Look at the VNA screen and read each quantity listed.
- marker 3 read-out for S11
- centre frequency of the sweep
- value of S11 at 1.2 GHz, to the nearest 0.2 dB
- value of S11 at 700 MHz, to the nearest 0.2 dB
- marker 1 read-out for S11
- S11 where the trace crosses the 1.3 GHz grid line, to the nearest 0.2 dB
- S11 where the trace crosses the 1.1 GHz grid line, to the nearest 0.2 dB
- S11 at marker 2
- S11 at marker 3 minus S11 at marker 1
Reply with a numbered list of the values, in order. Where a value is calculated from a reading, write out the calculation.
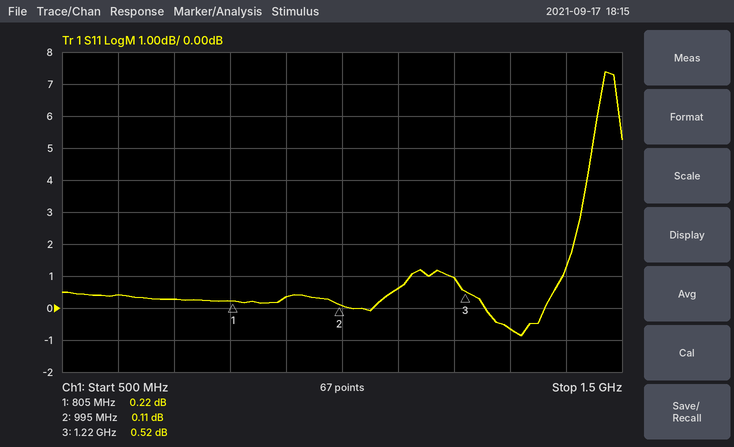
1. 0.52 dB
2. 1 GHz
3. 1.0 dB
4. 0.2 dB
5. 0.22 dB
6. -0.6 dB
7. 0.6 dB
8. 0.11 dB
9. 0.52 − (0.22) = 0.30 dB
